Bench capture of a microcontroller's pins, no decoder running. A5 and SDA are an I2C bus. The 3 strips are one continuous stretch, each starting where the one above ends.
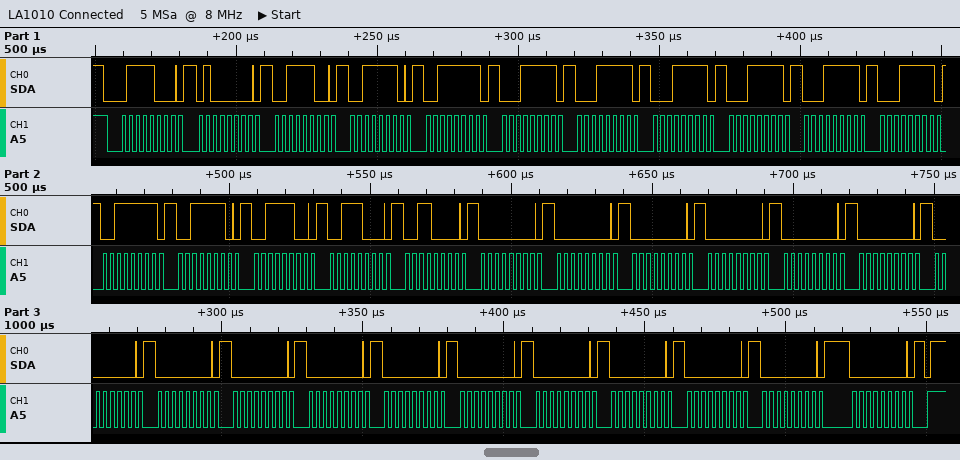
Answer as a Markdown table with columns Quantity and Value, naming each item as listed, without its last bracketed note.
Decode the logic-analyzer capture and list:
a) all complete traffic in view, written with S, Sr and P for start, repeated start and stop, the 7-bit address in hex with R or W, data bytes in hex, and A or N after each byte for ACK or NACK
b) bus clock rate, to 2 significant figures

| Quantity | Value |
|---|---|
| all complete traffic in view, written with S, Sr and P for start, repeated start and stop, the 7-bit address in hex with R or W, data bytes in hex, and A or N after each byte for ACK or NACK | S 3CW A 40 A 3C A 3E A 3F A 1F A 1F A 1F A 1F A 1F A 1F A 3F A 3E A 3C A 38 A 30 A 00 A 00 A 00 A 00 A 00 A 00 A 00 A 00 A 00 A 00 A 00 A 00 A 00 A 00 A 00 A 00 A 00 A P |
| bus clock rate, to 2 significant figures | 400 kHz |
